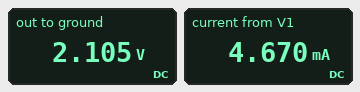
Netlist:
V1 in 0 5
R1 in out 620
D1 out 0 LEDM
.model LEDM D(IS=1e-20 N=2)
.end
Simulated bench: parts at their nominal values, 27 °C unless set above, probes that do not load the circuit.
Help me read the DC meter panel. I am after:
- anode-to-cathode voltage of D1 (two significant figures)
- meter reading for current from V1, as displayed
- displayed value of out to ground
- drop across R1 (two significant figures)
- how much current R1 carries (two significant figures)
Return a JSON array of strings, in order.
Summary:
["2.1 V", "4.670 mA", "2.105 V", "2.9 V", "4.7 mA"]
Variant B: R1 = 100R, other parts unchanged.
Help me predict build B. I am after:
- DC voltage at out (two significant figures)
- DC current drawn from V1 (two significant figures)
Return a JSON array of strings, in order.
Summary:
["2.2 V", "28 mA"]
